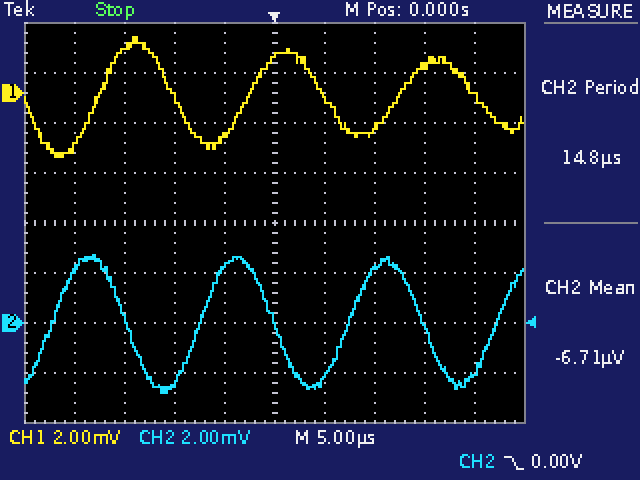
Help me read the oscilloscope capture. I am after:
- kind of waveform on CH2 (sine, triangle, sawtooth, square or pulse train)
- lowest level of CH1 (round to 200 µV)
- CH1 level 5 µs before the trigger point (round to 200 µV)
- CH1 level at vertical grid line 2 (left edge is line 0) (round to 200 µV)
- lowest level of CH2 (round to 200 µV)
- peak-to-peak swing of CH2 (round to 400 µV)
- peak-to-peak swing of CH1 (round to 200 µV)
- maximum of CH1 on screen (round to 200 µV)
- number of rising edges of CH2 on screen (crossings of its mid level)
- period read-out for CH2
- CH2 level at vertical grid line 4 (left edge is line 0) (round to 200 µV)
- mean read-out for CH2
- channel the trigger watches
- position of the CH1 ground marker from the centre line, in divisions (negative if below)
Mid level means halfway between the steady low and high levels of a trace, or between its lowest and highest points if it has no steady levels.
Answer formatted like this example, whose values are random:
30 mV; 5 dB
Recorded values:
sine; -2.6 mV; -1.8 mV; 1.8 mV; -2.8 mV; 5.6 mV; 4.8 mV; 2.2 mV; 4; 14.8 µs; 2.2 mV; -6.71 µV; CH2; +2.6 div
